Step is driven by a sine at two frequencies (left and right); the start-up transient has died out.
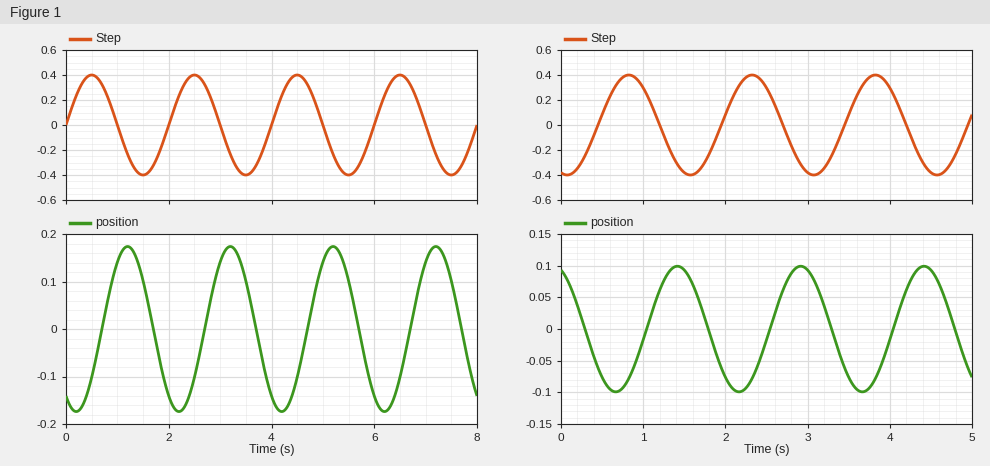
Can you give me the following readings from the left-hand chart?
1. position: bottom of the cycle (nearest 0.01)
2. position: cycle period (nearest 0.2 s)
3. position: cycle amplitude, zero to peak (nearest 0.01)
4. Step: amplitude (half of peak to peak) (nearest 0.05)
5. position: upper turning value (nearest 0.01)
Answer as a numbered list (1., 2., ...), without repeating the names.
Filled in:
1. -0.17
2. 2.0 s
3. 0.17
4. 0.40
5. 0.17
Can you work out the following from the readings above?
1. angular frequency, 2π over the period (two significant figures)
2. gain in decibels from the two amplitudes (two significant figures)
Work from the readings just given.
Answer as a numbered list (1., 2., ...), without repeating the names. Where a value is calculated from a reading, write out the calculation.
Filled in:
1. 2π / 2 = 3.1 rad/s
2. 20 log10(0.17 / 0.4) = -7.4 dB
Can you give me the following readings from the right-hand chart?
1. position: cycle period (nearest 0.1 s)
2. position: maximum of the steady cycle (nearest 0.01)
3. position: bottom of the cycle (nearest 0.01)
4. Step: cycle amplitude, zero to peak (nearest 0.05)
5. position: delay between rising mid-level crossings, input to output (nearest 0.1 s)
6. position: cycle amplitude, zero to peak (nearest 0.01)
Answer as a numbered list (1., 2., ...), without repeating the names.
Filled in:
1. 1.5 s
2. 0.10
3. -0.10
4. 0.40
5. 0.6 s
6. 0.10
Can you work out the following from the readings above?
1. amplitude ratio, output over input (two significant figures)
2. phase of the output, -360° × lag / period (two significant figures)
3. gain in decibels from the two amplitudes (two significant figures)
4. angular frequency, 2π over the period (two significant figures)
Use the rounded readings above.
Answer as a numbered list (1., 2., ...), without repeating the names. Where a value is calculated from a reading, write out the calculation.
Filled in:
1. 0.1 / 0.4 = 0.25
2. -360 × 0.6 / 1.5 = -140°
3. 20 log10(0.1 / 0.4) = -12 dB
4. 2π / 1.5 = 4.2 rad/s
